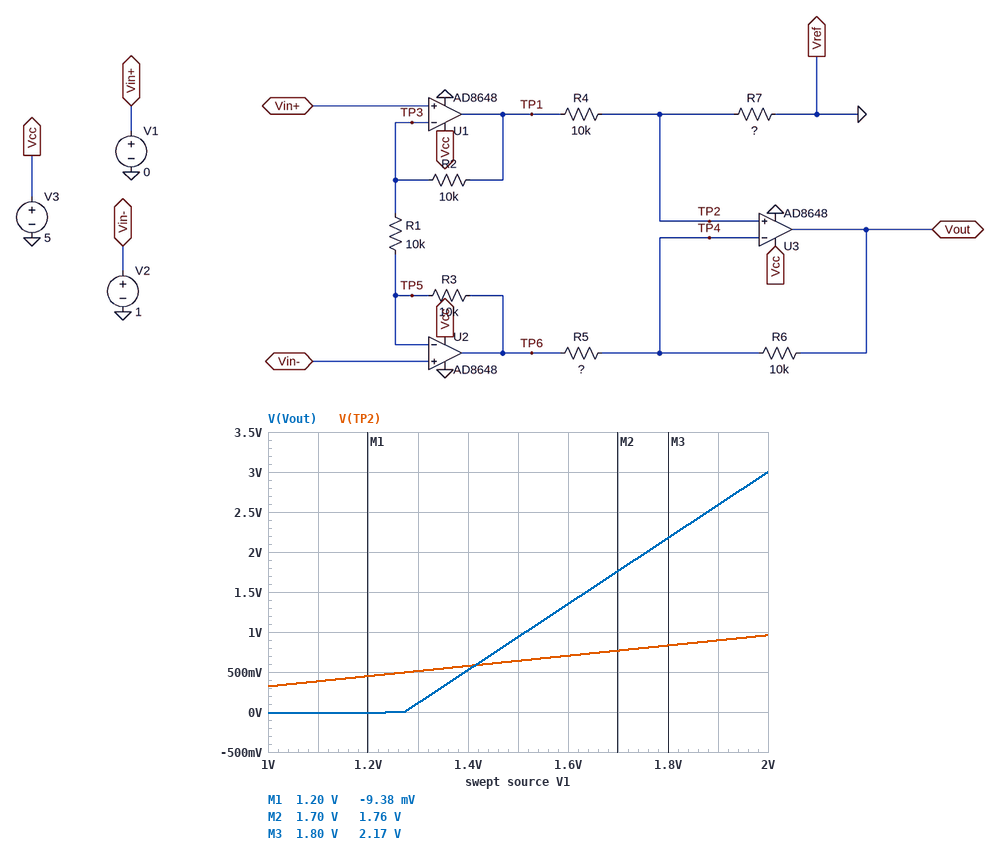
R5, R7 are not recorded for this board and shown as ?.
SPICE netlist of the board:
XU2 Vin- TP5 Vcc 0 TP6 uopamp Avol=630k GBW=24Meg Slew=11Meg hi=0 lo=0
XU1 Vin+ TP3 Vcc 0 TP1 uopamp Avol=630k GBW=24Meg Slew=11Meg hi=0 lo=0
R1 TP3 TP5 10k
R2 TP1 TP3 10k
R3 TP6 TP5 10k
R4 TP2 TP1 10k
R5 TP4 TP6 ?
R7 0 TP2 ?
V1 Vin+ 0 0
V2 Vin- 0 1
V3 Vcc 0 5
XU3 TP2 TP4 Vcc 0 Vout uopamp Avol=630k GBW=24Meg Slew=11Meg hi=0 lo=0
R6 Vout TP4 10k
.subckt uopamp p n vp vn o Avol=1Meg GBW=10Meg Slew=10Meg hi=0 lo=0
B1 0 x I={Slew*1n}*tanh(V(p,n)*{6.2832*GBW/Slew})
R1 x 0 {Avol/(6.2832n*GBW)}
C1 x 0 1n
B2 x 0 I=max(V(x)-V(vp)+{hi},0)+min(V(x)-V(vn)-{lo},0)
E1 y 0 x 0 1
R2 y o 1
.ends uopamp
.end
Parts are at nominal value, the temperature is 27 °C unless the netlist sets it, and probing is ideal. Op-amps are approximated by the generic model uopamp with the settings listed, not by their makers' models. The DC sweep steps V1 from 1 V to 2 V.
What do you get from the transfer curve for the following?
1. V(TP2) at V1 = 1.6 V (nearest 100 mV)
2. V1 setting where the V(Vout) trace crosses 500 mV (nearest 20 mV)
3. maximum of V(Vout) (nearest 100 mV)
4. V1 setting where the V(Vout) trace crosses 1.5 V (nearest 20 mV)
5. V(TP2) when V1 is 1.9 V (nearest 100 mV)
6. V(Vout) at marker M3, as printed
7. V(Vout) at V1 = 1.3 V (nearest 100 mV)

700 mV
1.40 V
3.0 V
1.64 V
900 mV
2.17 V
100 mV
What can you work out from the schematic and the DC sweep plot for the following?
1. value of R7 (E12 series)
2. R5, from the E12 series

4.7 kΩ
4.7 kΩ
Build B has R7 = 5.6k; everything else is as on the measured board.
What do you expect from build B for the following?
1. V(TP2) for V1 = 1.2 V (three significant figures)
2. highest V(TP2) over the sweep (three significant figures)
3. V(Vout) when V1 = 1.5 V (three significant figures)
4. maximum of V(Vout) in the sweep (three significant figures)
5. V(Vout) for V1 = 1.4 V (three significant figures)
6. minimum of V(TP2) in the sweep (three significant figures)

503 mV
1.08 V
1.18 V
3.37 V
744 mV
359 mV
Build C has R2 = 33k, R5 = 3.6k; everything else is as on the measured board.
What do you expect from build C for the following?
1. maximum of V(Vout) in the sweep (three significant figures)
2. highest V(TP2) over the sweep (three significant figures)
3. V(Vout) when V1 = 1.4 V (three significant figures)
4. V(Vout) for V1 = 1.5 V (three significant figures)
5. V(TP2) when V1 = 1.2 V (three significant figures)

5.01 V
1.60 V
1.62 V
2.42 V
595 mV
